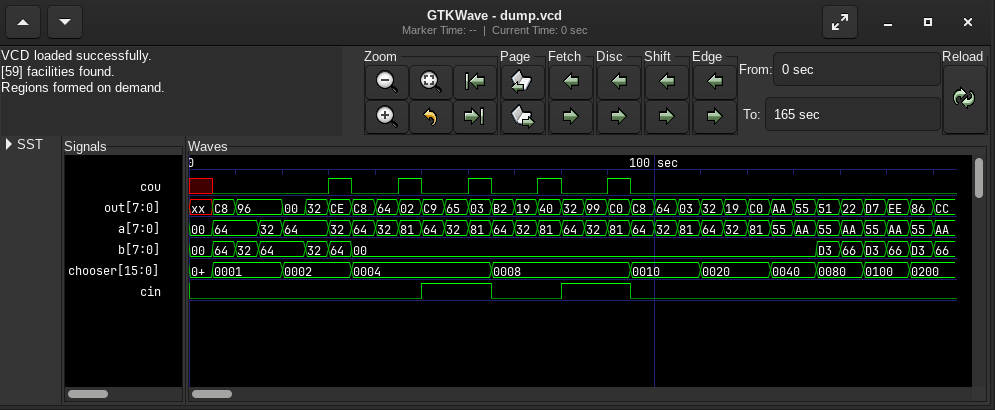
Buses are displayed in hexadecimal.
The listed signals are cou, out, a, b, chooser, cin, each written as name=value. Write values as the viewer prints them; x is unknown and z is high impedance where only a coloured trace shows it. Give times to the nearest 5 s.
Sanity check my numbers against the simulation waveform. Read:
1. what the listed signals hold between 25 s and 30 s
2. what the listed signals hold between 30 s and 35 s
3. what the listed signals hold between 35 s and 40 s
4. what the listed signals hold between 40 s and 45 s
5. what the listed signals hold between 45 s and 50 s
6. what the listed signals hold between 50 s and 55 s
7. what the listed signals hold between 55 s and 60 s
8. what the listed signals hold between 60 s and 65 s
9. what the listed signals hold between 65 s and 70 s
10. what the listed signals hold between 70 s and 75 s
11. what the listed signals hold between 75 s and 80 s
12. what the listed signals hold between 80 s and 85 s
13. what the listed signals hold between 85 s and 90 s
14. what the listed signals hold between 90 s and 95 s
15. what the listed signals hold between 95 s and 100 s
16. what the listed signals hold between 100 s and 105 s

cou=0, out=32, a=64, b=32, chooser=0002, cin=0
cou=1, out=CE, a=32, b=64, chooser=0002, cin=0
cou=0, out=C8, a=64, b=00, chooser=0004, cin=0
cou=0, out=64, a=32, b=00, chooser=0004, cin=0
cou=1, out=02, a=81, b=00, chooser=0004, cin=0
cou=0, out=C9, a=64, b=00, chooser=0004, cin=1
cou=0, out=65, a=32, b=00, chooser=0004, cin=1
cou=1, out=03, a=81, b=00, chooser=0004, cin=1
cou=0, out=B2, a=64, b=00, chooser=0008, cin=0
cou=0, out=19, a=32, b=00, chooser=0008, cin=0
cou=1, out=40, a=81, b=00, chooser=0008, cin=0
cou=0, out=32, a=64, b=00, chooser=0008, cin=1
cou=0, out=99, a=32, b=00, chooser=0008, cin=1
cou=1, out=C0, a=81, b=00, chooser=0008, cin=1
cou=0, out=C8, a=64, b=00, chooser=0010, cin=0
cou=0, out=64, a=32, b=00, chooser=0010, cin=0
